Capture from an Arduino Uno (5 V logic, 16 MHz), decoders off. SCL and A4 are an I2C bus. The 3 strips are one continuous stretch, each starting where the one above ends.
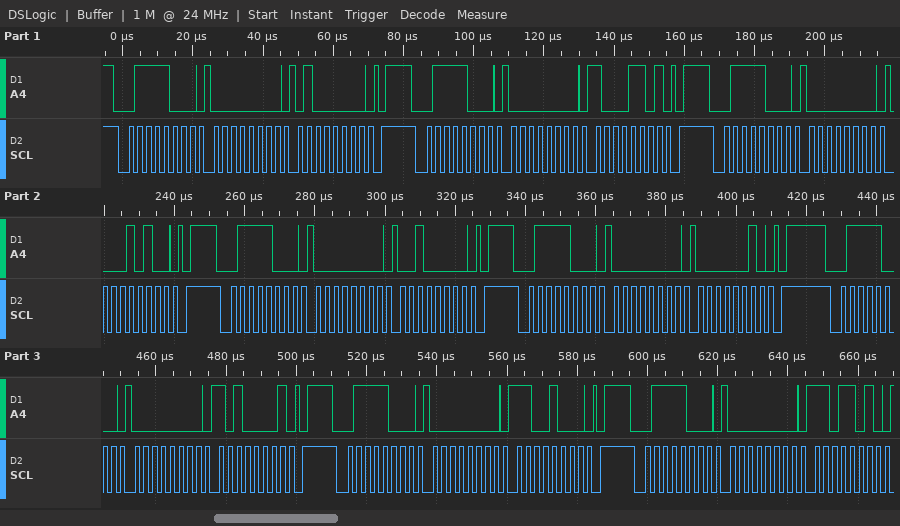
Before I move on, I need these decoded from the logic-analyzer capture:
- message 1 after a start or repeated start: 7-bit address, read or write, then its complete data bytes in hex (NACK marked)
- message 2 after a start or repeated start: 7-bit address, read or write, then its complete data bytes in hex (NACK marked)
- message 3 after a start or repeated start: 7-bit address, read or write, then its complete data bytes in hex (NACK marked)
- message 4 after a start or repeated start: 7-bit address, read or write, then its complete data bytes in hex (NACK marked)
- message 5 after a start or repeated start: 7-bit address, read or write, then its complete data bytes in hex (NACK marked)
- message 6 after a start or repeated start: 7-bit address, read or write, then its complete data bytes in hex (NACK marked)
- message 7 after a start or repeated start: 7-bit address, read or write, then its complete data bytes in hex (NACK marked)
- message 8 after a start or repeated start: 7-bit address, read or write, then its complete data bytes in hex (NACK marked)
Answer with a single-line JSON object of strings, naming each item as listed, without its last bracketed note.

{"message 1 after a start or repeated start: 7-bit address, read or write, then its complete data bytes in hex": "0x3C write: 00 40", "message 2 after a start or repeated start: 7-bit address, read or write, then its complete data bytes in hex": "0x3C write: 00 8D", "message 3 after a start or repeated start: 7-bit address, read or write, then its complete data bytes in hex": "0x3C write: 00 14", "message 4 after a start or repeated start: 7-bit address, read or write, then its complete data bytes in hex": "0x3C write: 00 20", "message 5 after a start or repeated start: 7-bit address, read or write, then its complete data bytes in hex": "0x3C write: 00 02", "message 6 after a start or repeated start: 7-bit address, read or write, then its complete data bytes in hex": "0x3C write: 00 A1", "message 7 after a start or repeated start: 7-bit address, read or write, then its complete data bytes in hex": "0x3C write: 00 C8", "message 8 after a start or repeated start: 7-bit address, read or write, then its complete data bytes in hex": "0x3C write: 00 DA"}
